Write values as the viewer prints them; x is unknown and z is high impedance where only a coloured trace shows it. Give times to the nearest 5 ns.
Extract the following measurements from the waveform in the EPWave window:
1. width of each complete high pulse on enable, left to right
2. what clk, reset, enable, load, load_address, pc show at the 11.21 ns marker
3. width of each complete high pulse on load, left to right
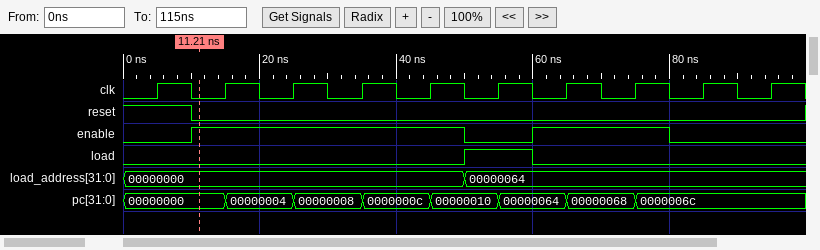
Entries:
40 ns, 20 ns
clk=0, reset=0, enable=1, load=0, load_address=00000000, pc=00000000
10 ns
